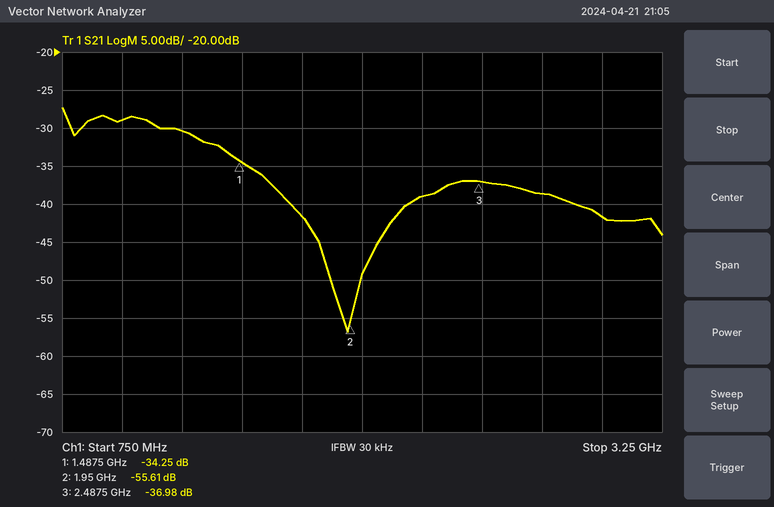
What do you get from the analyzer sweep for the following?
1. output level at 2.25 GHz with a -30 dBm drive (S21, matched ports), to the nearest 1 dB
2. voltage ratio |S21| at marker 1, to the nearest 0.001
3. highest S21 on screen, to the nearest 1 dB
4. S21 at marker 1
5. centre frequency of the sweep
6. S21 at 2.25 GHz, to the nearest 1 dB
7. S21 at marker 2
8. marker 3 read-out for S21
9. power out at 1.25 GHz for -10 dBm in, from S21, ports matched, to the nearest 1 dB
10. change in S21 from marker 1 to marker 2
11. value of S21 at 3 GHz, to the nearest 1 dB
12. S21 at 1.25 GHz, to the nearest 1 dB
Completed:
-69 dBm
0.019
-27 dB
-34.25 dB
2 GHz
-39 dB
-55.61 dB
-36.98 dB
-40 dBm
-21.36 dB
-42 dB
-30 dB
